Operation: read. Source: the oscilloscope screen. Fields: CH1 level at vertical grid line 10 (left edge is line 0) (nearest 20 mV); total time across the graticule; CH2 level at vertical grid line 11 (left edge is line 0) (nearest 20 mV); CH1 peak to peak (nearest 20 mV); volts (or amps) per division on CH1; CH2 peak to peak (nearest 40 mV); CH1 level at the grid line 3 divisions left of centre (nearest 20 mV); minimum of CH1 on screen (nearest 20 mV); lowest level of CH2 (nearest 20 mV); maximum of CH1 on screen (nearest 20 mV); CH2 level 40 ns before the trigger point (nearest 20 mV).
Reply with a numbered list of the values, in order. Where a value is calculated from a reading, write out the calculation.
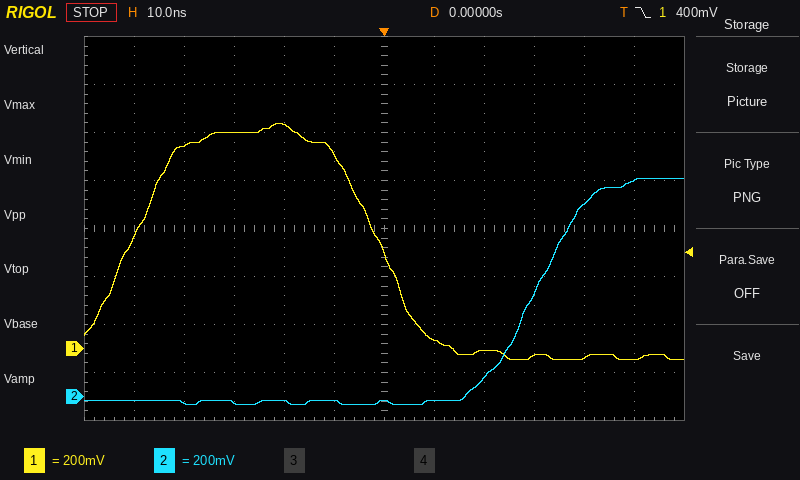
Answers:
1. -40 mV
2. 120 ns
3. 900 mV
4. 940 mV − (-40 mV) = 980 mV
5. 200 mV
6. 960 mV
7. 900 mV
8. -40 mV
9. -40 mV
10. 940 mV
11. -20 mV
